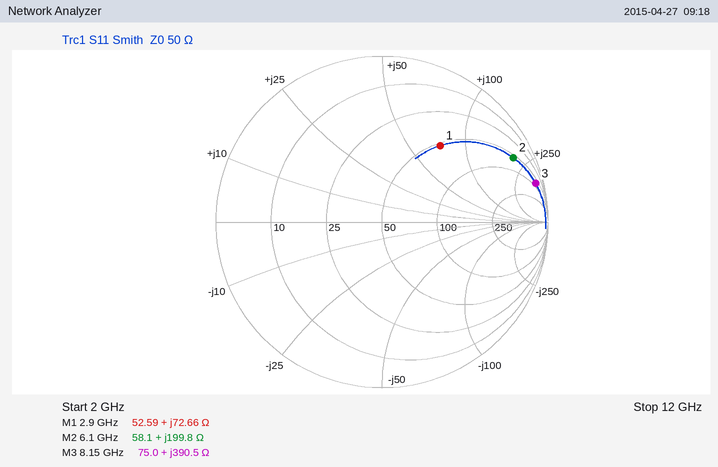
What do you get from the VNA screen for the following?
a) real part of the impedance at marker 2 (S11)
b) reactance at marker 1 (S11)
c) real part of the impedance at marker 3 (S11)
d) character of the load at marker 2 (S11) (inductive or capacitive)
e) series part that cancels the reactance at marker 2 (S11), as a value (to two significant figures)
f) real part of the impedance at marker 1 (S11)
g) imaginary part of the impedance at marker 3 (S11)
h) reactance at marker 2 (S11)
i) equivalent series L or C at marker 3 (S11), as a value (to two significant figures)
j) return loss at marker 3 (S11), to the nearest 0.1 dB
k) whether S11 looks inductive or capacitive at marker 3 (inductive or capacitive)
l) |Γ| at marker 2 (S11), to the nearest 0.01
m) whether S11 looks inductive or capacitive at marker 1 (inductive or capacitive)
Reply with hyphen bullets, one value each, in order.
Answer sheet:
- 58.1 Ω
- +72.66 Ω
- 75.0 Ω
- inductive
- 130 fF
- 52.59 Ω
- +390.5 Ω
- +199.8 Ω
- 7.6 nH
- 0.4 dB
- inductive
- 0.88
- inductive
